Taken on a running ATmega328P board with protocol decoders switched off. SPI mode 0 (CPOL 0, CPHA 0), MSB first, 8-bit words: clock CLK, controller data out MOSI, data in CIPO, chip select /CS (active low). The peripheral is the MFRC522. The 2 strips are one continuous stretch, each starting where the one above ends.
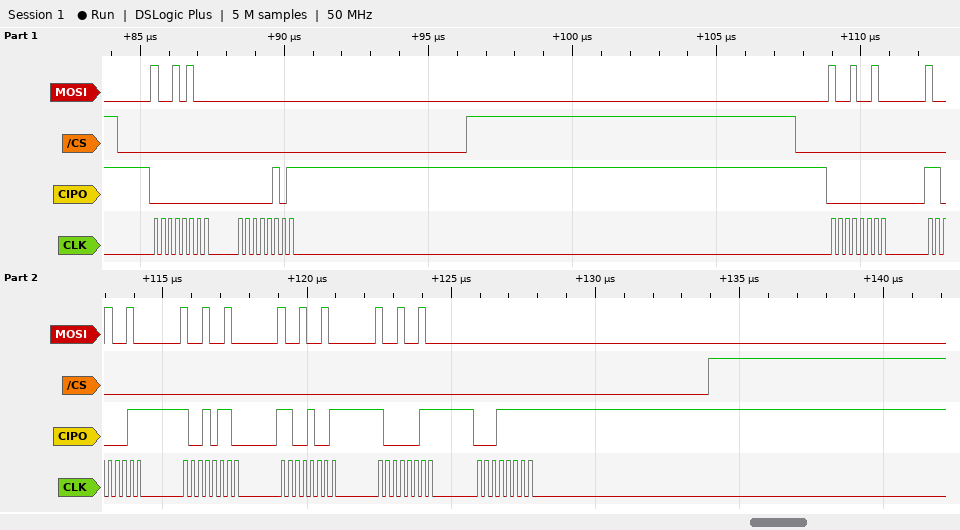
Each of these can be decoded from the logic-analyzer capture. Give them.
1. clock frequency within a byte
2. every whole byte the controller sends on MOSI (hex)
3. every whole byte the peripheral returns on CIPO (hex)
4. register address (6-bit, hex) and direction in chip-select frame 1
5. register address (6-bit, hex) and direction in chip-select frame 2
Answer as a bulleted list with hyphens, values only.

- 4 MHz
- 94 00 92 92 92 92 92 00
- 00 05 00 C3 96 C9 83 1F
- 0x0A read
- 0x09 read
